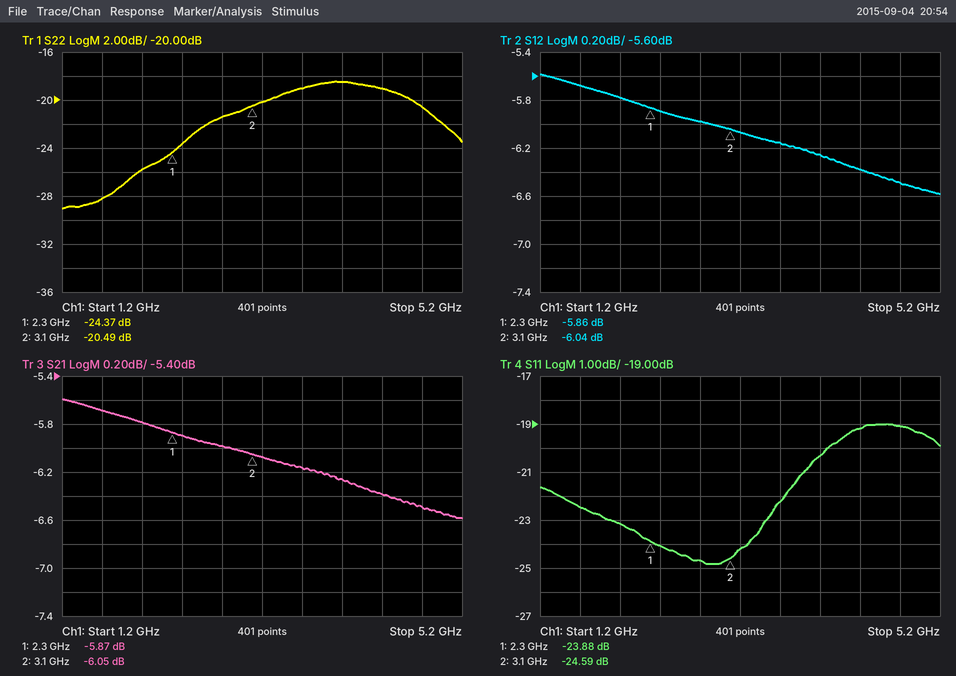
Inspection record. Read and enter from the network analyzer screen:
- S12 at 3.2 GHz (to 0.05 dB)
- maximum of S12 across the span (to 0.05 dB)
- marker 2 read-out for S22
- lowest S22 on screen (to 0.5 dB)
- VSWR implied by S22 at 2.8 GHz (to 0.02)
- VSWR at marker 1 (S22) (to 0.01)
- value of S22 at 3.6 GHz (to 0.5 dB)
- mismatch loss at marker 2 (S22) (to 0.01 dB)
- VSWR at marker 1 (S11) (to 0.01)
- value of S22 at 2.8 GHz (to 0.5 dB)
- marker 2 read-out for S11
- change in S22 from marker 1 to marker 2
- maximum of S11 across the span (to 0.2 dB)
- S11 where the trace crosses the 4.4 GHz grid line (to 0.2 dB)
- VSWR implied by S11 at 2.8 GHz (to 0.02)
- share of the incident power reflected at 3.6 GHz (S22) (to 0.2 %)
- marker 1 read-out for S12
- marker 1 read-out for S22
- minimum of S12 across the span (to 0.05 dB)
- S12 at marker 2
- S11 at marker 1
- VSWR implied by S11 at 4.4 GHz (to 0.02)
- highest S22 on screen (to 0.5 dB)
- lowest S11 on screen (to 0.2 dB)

-6.05 dB
-5.60 dB
-20.49 dB
-29.0 dB
1.18
1.13
-19.0 dB
0.04 dB
1.14
-21.5 dB
-24.59 dB
3.88 dB
-19.0 dB
-19.2 dB
1.12
1.2 %
-5.86 dB
-24.37 dB
-6.60 dB
-6.04 dB
-23.88 dB
1.24
-18.5 dB
-24.8 dB
